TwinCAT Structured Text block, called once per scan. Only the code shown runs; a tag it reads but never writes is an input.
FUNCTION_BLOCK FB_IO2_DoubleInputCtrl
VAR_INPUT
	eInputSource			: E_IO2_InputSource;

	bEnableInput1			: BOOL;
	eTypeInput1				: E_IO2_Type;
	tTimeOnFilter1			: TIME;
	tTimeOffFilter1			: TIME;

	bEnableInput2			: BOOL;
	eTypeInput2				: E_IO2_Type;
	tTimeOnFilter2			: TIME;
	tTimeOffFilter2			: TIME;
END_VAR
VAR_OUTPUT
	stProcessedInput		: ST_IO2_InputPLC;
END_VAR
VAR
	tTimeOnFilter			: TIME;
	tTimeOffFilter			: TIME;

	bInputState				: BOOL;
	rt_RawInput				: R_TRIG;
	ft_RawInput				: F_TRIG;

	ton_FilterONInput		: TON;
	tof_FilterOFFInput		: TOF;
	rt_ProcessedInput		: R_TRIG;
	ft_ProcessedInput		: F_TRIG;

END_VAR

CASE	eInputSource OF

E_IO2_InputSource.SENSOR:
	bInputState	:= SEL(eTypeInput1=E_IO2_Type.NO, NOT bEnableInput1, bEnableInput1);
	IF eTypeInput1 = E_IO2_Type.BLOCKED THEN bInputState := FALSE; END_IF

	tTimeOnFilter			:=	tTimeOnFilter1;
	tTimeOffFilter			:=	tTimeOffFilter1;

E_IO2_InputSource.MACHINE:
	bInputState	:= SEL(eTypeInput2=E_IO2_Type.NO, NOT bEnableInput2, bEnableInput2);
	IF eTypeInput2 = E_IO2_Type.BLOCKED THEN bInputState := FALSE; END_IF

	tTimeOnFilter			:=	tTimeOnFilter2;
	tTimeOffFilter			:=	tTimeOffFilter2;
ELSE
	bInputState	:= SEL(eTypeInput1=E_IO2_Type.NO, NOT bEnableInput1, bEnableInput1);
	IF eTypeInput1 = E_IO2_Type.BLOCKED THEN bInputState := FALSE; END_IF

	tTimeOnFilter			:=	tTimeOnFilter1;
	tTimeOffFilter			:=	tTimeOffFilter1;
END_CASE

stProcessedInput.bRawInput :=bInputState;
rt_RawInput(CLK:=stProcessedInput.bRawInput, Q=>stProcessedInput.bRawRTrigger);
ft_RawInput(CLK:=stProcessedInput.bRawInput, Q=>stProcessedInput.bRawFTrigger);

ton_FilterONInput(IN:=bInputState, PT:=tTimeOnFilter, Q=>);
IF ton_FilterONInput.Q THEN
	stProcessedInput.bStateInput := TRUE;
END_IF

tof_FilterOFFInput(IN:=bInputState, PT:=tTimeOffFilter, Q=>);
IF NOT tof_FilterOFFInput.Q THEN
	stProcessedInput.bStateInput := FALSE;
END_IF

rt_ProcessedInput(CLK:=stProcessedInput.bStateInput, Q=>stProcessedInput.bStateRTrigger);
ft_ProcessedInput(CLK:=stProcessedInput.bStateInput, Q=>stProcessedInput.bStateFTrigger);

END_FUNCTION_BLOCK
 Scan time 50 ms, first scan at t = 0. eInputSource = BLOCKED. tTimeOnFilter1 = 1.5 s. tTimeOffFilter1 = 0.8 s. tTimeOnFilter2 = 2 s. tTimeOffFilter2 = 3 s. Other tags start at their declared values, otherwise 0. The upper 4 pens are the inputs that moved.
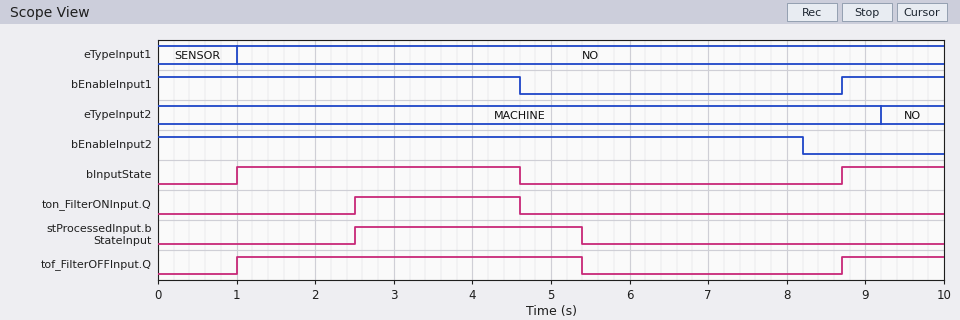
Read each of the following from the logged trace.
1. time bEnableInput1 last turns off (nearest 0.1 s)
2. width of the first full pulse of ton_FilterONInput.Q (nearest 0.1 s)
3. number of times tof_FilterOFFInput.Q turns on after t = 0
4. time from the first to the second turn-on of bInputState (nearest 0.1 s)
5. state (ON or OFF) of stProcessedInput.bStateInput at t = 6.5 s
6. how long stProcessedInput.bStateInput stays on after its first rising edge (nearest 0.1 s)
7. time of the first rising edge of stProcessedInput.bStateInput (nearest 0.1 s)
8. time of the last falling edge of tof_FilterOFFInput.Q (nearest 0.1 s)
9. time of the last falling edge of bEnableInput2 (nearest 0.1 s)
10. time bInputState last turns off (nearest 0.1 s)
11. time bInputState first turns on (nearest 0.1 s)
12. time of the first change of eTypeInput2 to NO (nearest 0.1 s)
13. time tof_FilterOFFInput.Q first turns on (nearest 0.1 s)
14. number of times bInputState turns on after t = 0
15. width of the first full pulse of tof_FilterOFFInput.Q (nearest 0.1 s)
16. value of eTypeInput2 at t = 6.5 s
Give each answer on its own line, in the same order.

4.6 s
2.1 s
2
7.7 s
OFF
2.9 s
2.5 s
5.4 s
8.2 s
4.6 s
1.0 s
9.2 s
1.0 s
2
4.4 s
MACHINE
